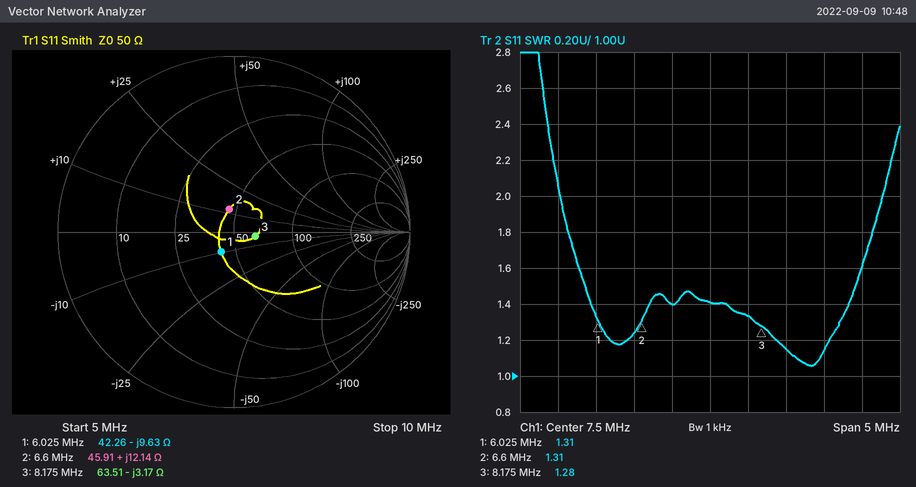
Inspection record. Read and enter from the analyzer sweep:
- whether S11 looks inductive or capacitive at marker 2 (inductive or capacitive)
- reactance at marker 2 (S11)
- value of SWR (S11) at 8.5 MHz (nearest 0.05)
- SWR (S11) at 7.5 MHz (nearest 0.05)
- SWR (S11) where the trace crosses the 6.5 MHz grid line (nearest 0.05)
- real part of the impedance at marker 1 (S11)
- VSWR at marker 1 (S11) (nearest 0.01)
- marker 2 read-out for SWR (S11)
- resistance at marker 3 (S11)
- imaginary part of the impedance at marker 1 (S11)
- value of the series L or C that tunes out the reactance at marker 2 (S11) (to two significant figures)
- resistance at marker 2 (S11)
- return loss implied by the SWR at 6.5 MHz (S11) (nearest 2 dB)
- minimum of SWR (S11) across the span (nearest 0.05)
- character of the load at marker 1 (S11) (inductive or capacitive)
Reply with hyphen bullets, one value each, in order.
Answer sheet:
- inductive
- +12.14 Ω
- 1.15
- 1.40
- 1.25
- 42.26 Ω
- 1.31
- 1.31
- 63.51 Ω
- -9.63 Ω
- 2.0 nF
- 45.91 Ω
- 20 dB
- 1.05
- capacitive
